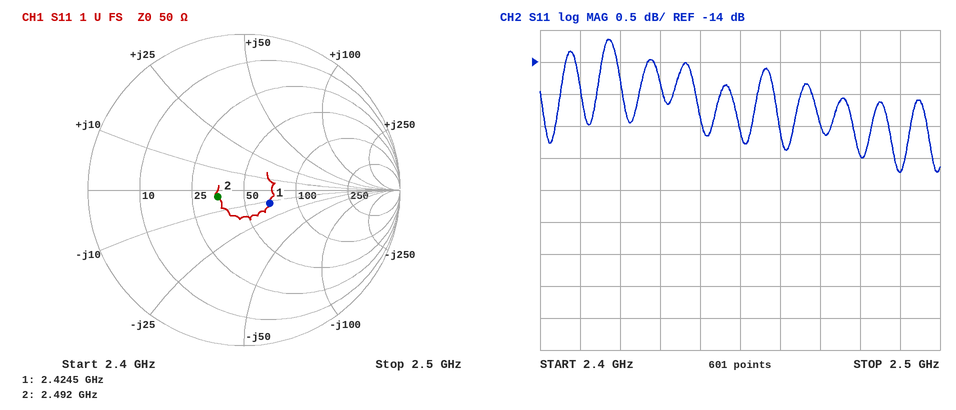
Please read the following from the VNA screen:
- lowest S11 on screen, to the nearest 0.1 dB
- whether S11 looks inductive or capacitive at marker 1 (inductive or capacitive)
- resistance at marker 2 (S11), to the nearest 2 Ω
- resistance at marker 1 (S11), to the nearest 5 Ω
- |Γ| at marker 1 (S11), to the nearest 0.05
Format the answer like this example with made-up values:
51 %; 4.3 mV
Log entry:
-15.7 dB; capacitive; 36 Ω; 70 Ω; 0.20
